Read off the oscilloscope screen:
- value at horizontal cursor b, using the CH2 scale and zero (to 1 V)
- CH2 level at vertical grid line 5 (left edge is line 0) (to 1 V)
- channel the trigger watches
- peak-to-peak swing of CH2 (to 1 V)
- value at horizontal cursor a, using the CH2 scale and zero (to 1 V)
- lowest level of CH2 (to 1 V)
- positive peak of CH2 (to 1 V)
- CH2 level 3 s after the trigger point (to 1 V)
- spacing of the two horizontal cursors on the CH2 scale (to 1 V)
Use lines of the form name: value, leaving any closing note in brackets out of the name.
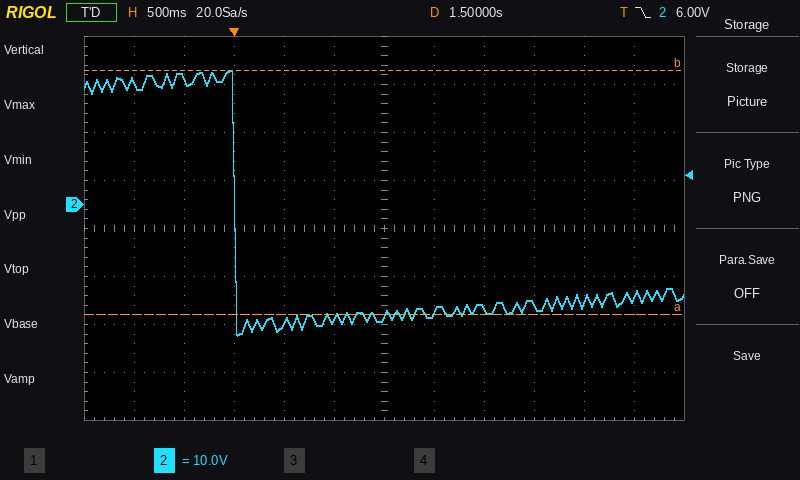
value at horizontal cursor b, using the CH2 scale and zero: 28 V
CH2 level at vertical grid line 5 (left edge is line 0): -24 V
channel the trigger watches: CH2
peak-to-peak swing of CH2: 55 V
value at horizontal cursor a, using the CH2 scale and zero: -23 V
lowest level of CH2: -27 V
positive peak of CH2: 28 V
CH2 level 3 s after the trigger point: -21 V
spacing of the two horizontal cursors on the CH2 scale: 51 V
